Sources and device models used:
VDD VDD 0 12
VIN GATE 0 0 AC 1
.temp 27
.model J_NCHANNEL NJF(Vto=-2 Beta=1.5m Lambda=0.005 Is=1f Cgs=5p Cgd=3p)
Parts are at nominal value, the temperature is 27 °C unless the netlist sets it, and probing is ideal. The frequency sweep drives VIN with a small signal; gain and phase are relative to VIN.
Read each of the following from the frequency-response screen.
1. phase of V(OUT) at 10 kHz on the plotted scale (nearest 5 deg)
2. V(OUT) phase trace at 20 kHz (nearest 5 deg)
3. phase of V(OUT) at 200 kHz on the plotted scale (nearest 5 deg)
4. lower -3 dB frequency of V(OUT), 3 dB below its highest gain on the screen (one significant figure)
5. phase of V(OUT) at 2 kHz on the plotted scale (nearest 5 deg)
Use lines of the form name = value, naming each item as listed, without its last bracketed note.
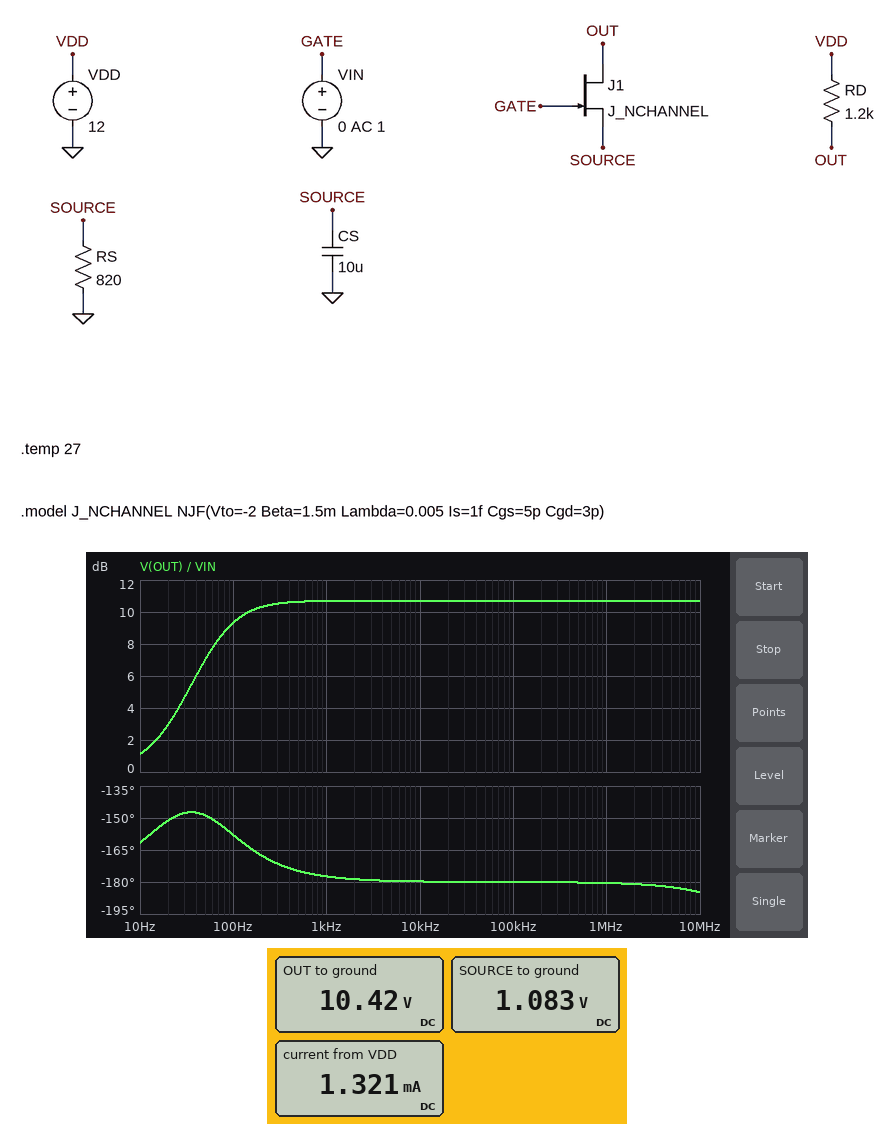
phase of V(OUT) at 10 kHz on the plotted scale = -180 deg
V(OUT) phase trace at 20 kHz = -180 deg
phase of V(OUT) at 200 kHz on the plotted scale = -180 deg
lower -3 dB frequency of V(OUT), 3 dB below its highest gain on the screen = 60 Hz
phase of V(OUT) at 2 kHz on the plotted scale = -180 deg
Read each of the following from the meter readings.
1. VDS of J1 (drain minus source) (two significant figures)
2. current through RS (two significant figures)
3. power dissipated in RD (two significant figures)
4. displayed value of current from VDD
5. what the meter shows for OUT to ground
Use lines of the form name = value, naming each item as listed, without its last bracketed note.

VDS of J1 (drain minus source) = 9.3 V
current through RS = 1.3 mA
power dissipated in RD = 2.1 mW
displayed value of current from VDD = 1.321 mA
what the meter shows for OUT to ground = 10.42 V
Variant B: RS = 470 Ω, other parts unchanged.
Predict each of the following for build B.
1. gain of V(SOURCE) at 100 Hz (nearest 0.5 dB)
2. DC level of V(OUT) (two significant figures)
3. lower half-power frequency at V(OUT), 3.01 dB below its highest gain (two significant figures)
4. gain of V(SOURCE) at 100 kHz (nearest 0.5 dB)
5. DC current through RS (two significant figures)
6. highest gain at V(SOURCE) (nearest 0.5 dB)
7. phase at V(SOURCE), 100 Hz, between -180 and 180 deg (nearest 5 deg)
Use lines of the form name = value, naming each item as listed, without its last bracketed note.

gain of V(SOURCE) at 100 Hz = -8.0 dB
DC level of V(OUT) = 9.7 V
lower half-power frequency at V(OUT), 3.01 dB below its highest gain = 74 Hz
gain of V(SOURCE) at 100 kHz = -65.5 dB
DC current through RS = 1.9 mA
highest gain at V(SOURCE) = -4.0 dB
phase at V(SOURCE), 100 Hz, between -180 and 180 deg = -50 deg
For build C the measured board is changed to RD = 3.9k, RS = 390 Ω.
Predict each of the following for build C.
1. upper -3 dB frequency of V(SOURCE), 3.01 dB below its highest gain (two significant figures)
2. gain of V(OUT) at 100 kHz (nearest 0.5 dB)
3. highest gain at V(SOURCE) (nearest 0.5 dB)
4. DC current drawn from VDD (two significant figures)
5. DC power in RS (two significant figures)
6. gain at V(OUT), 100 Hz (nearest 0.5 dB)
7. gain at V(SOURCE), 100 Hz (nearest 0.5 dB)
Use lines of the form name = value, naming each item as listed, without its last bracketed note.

upper -3 dB frequency of V(SOURCE), 3.01 dB below its highest gain = 96 Hz
gain of V(OUT) at 100 kHz = 22.5 dB
highest gain at V(SOURCE) = -5.0 dB
DC current drawn from VDD = 2.1 mA
DC power in RS = 1.7 mW
gain at V(OUT), 100 Hz = 20.5 dB
gain at V(SOURCE), 100 Hz = -8.0 dB
